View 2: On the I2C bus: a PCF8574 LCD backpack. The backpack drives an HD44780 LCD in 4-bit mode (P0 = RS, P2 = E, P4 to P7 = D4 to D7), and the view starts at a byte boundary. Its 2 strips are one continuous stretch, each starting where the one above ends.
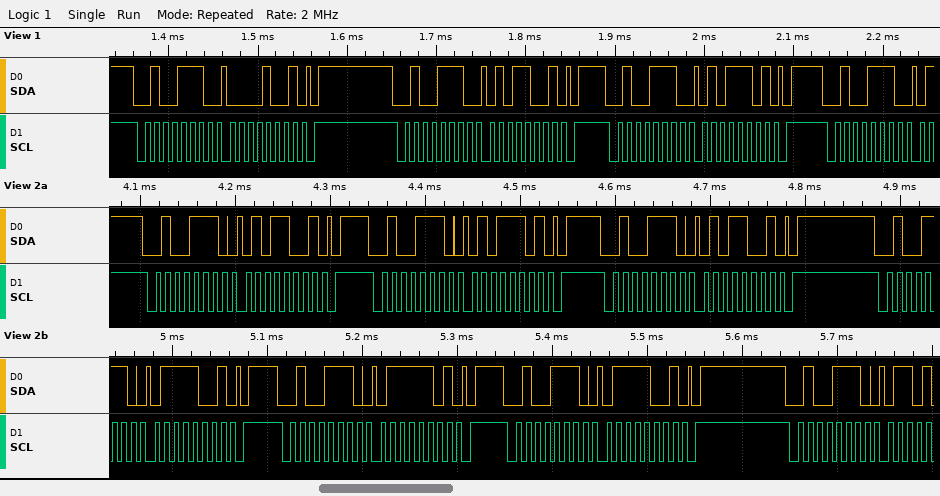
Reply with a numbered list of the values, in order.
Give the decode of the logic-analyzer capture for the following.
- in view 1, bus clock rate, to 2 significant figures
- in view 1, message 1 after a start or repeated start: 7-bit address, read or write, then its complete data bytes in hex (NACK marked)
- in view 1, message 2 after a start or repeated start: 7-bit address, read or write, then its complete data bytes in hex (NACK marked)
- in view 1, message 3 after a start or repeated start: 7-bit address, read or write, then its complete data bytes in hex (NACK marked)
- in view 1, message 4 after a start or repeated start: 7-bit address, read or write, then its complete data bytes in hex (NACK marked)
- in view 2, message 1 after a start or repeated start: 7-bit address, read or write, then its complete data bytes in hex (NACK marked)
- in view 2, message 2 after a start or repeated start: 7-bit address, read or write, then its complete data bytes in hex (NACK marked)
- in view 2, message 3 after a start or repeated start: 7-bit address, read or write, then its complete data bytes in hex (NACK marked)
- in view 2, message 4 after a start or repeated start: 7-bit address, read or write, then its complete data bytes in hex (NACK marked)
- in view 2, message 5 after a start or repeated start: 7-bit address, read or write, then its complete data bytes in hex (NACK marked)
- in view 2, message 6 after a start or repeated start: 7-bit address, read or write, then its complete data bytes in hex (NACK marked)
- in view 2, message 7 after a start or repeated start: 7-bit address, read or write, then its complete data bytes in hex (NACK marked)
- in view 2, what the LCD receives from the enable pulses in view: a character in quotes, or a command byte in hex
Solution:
1. 100 kHz
2. 0x27 write: 09
3. 0x27 write: 59
4. 0x27 write: 5D
5. 0x27 write
6. 0x27 write: 59
7. 0x27 write: 5D
8. 0x27 write: 59
9. 0x27 write: 79
10. 0x27 write: 7D
11. 0x27 write: 79
12. 0x27 write
13. 'W'
